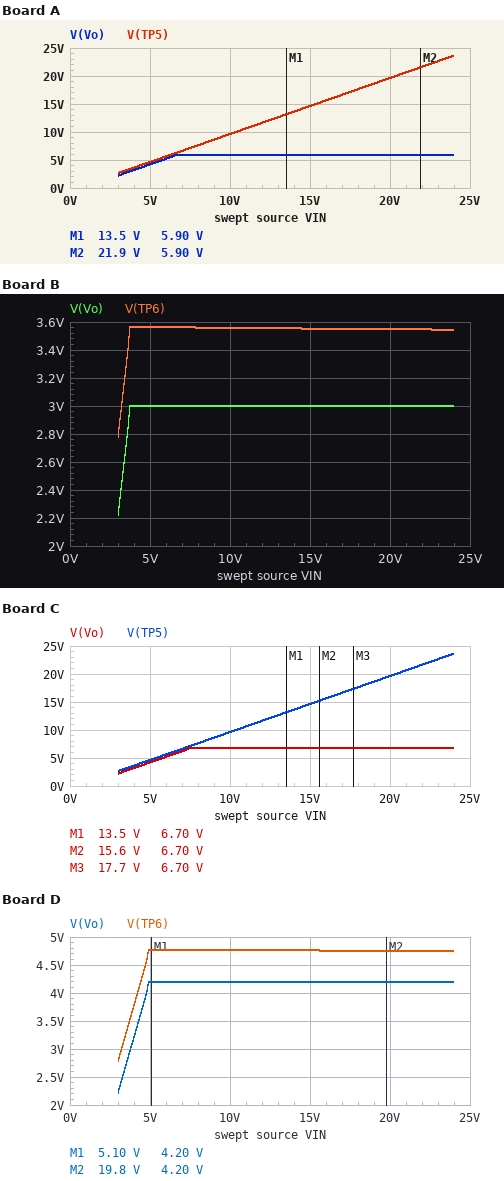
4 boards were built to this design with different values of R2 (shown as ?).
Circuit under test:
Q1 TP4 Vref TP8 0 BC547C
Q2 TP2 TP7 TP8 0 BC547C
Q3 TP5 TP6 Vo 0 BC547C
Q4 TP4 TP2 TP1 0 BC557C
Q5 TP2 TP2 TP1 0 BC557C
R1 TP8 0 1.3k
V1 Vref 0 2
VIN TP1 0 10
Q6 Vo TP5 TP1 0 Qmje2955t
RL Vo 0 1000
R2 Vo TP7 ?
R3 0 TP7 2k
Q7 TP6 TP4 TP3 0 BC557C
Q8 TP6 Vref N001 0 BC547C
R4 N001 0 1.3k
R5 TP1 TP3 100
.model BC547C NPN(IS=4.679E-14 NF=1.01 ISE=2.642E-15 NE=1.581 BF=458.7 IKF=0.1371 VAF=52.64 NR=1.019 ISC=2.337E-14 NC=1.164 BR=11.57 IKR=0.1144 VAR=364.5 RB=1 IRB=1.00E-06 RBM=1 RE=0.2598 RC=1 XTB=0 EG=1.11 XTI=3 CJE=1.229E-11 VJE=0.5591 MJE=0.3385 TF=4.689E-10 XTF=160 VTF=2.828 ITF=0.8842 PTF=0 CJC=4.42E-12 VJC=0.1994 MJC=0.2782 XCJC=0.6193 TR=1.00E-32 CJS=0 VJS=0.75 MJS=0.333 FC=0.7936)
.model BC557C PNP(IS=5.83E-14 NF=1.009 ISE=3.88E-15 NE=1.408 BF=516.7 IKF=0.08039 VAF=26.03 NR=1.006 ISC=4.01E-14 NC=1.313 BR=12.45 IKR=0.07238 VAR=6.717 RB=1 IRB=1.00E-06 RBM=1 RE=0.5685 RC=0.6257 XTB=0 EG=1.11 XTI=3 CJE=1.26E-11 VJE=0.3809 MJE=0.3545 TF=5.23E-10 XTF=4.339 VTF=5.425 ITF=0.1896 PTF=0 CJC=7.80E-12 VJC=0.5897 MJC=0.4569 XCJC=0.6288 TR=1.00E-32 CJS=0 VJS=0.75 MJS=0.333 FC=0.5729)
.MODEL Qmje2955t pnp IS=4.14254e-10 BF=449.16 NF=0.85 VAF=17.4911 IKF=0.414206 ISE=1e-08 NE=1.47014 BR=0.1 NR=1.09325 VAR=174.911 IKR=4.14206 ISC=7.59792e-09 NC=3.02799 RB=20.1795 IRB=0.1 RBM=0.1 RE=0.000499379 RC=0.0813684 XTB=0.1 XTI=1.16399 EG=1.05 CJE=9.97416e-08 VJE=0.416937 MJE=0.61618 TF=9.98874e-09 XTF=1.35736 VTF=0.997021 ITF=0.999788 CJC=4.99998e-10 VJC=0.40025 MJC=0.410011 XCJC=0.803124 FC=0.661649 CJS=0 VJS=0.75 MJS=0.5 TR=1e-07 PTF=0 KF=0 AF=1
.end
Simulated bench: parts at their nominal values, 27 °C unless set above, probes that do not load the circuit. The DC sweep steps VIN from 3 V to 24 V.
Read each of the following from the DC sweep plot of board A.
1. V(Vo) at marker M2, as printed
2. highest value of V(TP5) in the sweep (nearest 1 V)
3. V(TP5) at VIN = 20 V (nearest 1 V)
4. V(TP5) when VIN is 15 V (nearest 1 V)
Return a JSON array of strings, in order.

["5.90 V", "24 V", "20 V", "15 V"]
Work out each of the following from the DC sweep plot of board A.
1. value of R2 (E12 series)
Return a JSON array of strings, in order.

["3.9 kΩ"]
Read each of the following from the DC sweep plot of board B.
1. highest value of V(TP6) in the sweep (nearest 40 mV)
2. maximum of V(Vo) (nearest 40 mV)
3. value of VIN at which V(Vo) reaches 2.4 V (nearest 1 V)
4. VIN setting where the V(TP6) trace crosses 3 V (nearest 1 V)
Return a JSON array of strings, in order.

["3.56 V", "3.00 V", "3 V", "3 V"]
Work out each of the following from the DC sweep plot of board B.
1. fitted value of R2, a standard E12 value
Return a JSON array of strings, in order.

["1 kΩ"]
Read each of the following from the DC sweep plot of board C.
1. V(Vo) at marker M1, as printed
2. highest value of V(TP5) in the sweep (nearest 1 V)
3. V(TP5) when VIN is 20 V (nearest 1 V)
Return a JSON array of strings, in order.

["6.70 V", "24 V", "20 V"]
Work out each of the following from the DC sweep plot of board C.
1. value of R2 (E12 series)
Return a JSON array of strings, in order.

["4.7 kΩ"]
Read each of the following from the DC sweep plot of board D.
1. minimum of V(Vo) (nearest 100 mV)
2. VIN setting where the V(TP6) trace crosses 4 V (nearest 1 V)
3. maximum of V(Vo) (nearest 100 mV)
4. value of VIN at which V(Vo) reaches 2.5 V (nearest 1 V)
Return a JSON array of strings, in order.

["2.2 V", "4 V", "4.2 V", "3 V"]
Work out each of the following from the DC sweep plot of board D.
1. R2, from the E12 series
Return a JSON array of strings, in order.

["2.2 kΩ"]
